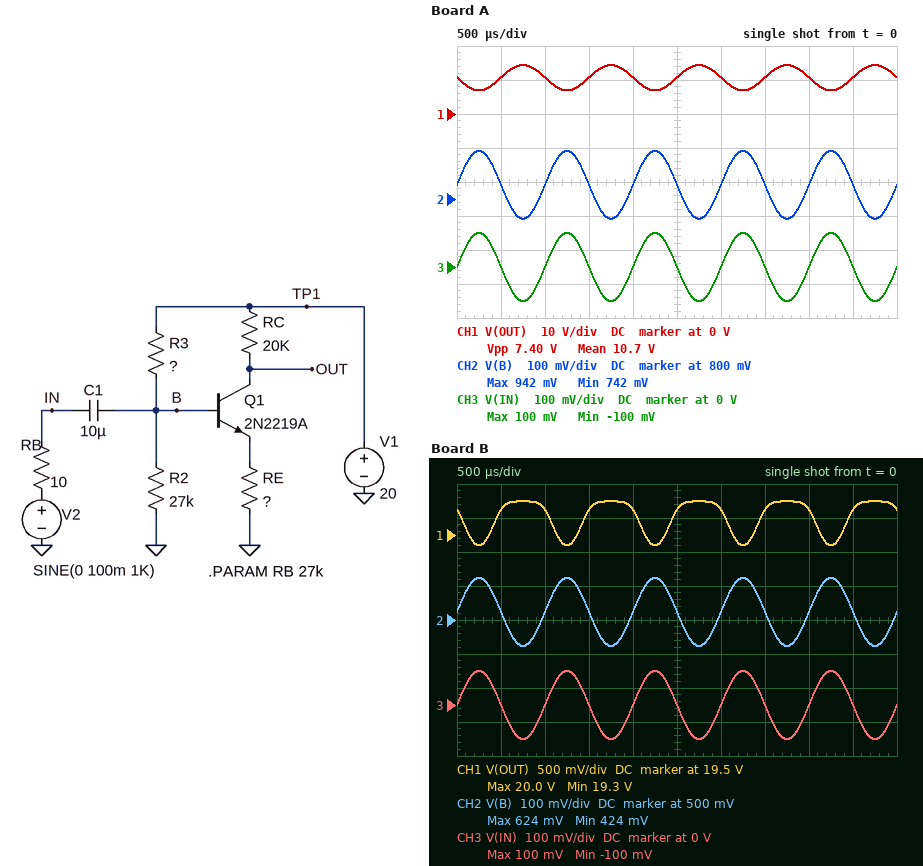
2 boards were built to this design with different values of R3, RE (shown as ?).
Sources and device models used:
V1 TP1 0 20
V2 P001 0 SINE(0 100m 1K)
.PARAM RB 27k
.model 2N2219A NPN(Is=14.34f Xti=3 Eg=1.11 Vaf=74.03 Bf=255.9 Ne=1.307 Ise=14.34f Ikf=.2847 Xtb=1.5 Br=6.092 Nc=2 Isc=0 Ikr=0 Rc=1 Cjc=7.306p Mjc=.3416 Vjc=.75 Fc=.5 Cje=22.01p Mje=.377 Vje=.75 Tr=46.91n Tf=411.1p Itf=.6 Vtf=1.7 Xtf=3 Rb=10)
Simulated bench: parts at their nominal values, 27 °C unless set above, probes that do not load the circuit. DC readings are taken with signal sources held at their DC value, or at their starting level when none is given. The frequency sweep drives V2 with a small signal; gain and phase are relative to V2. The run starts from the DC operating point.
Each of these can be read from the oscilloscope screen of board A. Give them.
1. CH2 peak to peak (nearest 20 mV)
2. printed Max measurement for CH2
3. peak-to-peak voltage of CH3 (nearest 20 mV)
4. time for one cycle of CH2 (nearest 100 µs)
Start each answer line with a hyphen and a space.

- 200 mV
- 942 mV
- 200 mV
- 1.0 ms
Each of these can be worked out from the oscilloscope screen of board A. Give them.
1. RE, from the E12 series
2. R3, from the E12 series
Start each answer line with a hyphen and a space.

- 470 Ω
- 560 kΩ
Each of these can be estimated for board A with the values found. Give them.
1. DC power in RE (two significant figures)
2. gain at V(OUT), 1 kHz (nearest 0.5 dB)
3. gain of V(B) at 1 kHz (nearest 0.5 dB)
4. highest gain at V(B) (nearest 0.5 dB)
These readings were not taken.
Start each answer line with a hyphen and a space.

- 100 µW
- 31.5 dB
- 0 dB
- 0 dB
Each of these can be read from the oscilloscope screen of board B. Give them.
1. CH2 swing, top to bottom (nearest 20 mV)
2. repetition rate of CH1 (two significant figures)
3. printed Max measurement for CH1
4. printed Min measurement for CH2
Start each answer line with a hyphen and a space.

- 200 mV
- 1.0 kHz
- 20.0 V
- 424 mV
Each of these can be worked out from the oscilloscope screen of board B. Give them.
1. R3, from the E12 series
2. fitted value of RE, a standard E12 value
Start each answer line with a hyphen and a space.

- 1 MΩ
- 2.2 kΩ
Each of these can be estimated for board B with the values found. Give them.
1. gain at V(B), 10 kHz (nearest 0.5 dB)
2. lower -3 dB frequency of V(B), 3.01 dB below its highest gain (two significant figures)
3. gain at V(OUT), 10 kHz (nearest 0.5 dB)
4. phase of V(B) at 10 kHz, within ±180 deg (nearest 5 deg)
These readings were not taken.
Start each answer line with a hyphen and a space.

- 0 dB
- 630 mHz
- 10.0 dB
- 0 deg
